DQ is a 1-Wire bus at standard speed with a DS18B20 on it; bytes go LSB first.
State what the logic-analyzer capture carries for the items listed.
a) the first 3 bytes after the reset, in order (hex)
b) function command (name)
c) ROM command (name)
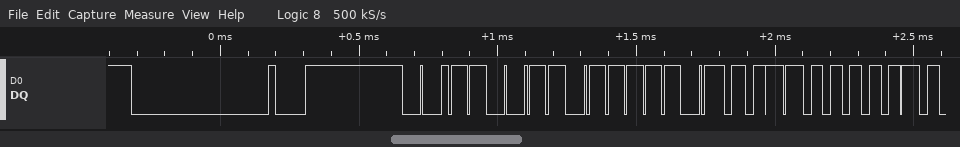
CC BE 0C
Read Scratchpad
Skip ROM
